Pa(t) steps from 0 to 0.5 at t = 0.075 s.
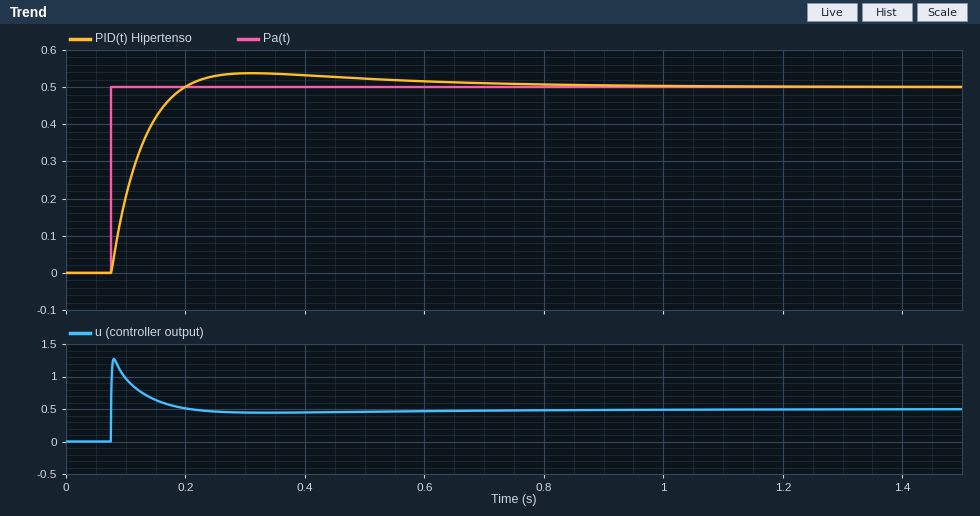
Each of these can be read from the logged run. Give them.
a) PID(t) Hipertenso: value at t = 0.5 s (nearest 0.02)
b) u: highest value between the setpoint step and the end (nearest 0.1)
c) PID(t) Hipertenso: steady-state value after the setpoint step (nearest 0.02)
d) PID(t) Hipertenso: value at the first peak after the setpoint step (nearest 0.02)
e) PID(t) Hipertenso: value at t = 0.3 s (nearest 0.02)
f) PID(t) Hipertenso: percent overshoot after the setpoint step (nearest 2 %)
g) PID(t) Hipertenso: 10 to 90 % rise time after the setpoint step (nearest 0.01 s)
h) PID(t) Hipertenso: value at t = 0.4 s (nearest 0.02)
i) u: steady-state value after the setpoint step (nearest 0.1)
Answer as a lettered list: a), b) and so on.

a) 0.52
b) 1.3
c) 0.50
d) 0.54
e) 0.54
f) 8 %
g) 0.08 s
h) 0.54
i) 0.5
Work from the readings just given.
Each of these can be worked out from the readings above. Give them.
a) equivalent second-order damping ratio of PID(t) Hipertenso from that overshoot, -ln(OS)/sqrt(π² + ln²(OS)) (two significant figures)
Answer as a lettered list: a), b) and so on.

a) 0.63
